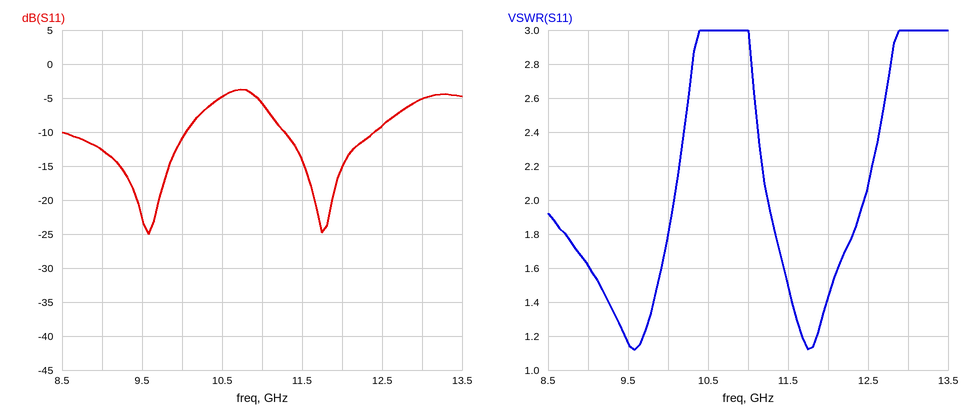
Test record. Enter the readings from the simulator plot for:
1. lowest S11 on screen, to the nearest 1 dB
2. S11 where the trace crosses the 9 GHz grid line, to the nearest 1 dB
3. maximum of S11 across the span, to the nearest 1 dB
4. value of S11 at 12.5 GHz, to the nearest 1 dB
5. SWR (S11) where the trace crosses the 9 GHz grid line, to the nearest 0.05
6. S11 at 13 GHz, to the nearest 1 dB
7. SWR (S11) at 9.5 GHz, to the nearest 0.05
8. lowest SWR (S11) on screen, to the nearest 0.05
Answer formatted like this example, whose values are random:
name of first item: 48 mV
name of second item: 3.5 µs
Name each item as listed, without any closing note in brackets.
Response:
lowest S11 on screen, to the nearest 1 dB: -25 dB
S11 where the trace crosses the 9 GHz grid line, to the nearest 1 dB: -13 dB
maximum of S11 across the span, to the nearest 1 dB: -4 dB
value of S11 at 12.5 GHz, to the nearest 1 dB: -9 dB
SWR (S11) where the trace crosses the 9 GHz grid line, to the nearest 0.05: 1.60
S11 at 13 GHz, to the nearest 1 dB: -5 dB
SWR (S11) at 9.5 GHz, to the nearest 0.05: 1.15
lowest SWR (S11) on screen, to the nearest 0.05: 1.10
